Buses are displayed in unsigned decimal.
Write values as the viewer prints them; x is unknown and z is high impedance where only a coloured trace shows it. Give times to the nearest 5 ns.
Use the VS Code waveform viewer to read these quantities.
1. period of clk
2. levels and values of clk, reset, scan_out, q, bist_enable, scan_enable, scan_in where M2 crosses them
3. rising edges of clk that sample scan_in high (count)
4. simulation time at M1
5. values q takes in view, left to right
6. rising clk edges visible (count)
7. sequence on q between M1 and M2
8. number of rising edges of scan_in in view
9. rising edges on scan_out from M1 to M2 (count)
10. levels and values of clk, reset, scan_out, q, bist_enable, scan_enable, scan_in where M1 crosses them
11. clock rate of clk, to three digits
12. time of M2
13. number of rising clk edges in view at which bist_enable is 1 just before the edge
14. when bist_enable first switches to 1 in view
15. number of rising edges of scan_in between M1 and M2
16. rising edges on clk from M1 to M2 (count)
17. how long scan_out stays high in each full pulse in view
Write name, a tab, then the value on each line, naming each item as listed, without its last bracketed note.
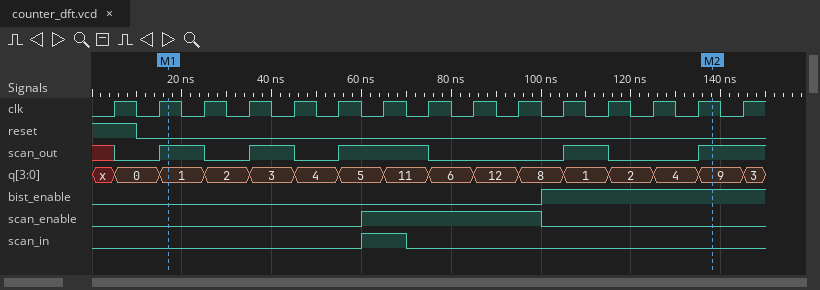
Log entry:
period of clk	10 ns
levels and values of clk, reset, scan_out, q, bist_enable, scan_enable, scan_in where M2 crosses them	clk=1, reset=0, scan_out=1, q=9, bist_enable=1, scan_enable=0, scan_in=0
rising edges of clk that sample scan_in high	1
simulation time at M1	15 ns
values q takes in view, left to right	x, 0, 1, 2, 3, 4, 5, 11, 6, 12, 8, 1, 2, 4, 9, 3
rising clk edges visible	15
sequence on q between M1 and M2	1, 2, 3, 4, 5, 11, 6, 12, 8, 1, 2, 4, 9
number of rising edges of scan_in in view	1
rising edges on scan_out from M1 to M2	4
levels and values of clk, reset, scan_out, q, bist_enable, scan_enable, scan_in where M1 crosses them	clk=1, reset=0, scan_out=1, q=1, bist_enable=0, scan_enable=0, scan_in=0
clock rate of clk, to three digits	100 MHz
time of M2	140 ns
number of rising clk edges in view at which bist_enable is 1 just before the edge	5
when bist_enable first switches to 1 in view	100 ns
number of rising edges of scan_in between M1 and M2	1
rising edges on clk from M1 to M2	12
how long scan_out stays high in each full pulse in view	10 ns, 10 ns, 20 ns, 10 ns
